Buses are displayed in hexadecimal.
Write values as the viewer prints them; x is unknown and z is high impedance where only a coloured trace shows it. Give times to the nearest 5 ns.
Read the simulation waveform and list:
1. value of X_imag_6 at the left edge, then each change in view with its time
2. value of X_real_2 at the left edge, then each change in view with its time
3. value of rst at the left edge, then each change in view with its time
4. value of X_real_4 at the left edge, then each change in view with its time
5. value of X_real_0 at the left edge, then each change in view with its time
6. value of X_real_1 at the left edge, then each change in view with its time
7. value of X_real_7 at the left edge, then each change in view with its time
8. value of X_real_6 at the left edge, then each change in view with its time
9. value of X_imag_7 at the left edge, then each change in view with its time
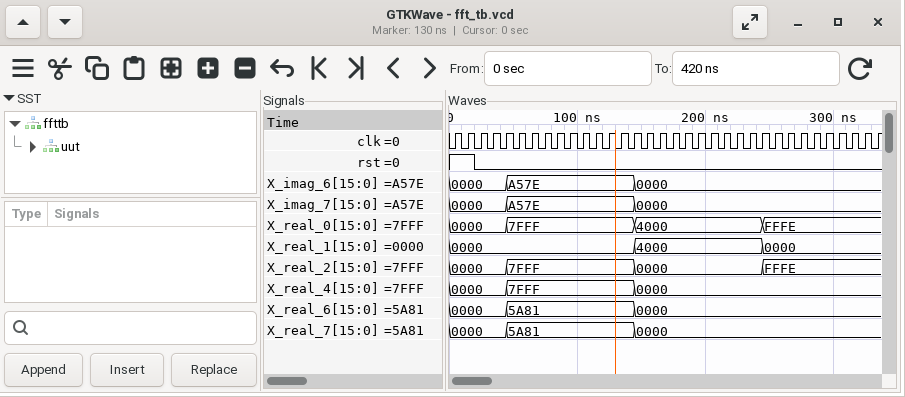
0000, A57E at 45 ns, 0000 at 145 ns
0000, 7FFF at 45 ns, 0000 at 145 ns, FFFE at 245 ns
1, 0 at 20 ns
0000, 7FFF at 45 ns, 0000 at 145 ns
0000, 7FFF at 45 ns, 4000 at 145 ns, FFFE at 245 ns
0000, 4000 at 145 ns, 0000 at 245 ns
0000, 5A81 at 45 ns, 0000 at 145 ns
0000, 5A81 at 45 ns, 0000 at 145 ns
0000, A57E at 45 ns, 0000 at 145 ns
